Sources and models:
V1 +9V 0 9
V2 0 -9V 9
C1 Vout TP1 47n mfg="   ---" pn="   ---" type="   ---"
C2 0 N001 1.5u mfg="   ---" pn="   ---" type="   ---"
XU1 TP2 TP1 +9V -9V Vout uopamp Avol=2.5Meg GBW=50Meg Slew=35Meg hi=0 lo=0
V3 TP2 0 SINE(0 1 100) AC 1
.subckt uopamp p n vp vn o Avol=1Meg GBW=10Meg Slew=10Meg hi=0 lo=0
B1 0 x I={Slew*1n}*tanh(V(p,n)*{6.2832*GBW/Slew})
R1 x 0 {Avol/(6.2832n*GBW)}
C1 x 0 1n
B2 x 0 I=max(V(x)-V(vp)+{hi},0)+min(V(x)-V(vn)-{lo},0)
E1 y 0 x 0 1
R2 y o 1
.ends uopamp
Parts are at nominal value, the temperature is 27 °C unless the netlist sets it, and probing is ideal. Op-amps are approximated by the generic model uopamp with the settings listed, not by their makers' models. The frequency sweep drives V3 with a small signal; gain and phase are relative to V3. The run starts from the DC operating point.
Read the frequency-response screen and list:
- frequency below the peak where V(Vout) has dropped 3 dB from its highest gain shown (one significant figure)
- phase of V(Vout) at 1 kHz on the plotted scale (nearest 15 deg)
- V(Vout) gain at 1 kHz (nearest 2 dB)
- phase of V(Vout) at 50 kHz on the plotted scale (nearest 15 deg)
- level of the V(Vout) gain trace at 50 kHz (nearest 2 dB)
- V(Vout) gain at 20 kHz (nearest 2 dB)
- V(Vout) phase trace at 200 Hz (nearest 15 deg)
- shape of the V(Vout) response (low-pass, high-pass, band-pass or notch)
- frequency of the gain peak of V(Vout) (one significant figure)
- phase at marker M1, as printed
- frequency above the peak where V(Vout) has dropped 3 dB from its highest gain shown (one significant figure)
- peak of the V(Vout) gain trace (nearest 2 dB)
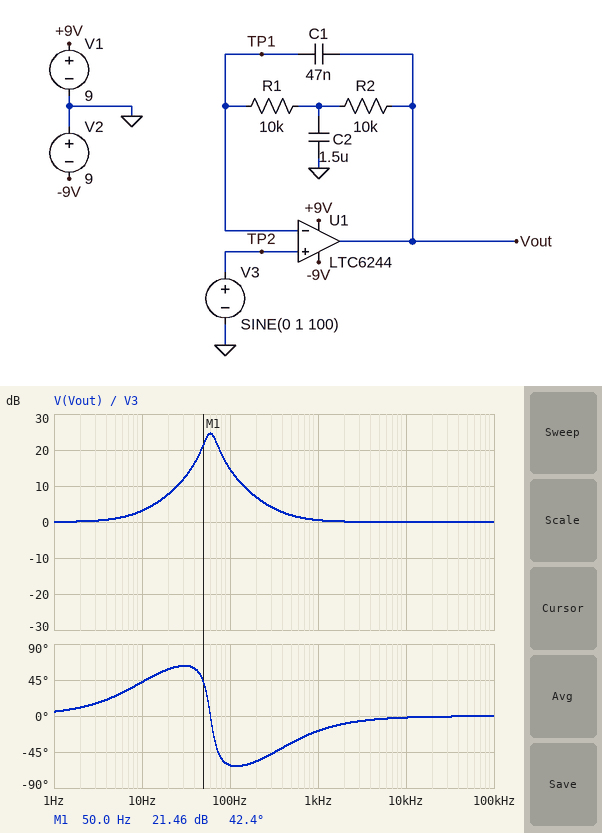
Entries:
50 Hz
-15 deg
0 dB
0 deg
0 dB
0 dB
-60 deg
band-pass
60 Hz
42.4 deg
70 Hz
24 dB
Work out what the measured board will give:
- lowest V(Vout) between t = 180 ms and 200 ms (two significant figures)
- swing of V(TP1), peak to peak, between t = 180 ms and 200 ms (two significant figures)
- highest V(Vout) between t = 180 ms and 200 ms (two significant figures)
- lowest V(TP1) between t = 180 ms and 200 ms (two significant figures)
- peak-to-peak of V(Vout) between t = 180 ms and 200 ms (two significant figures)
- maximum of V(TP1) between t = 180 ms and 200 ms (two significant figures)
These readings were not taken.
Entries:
-5.4 V
2.0 V
5.4 V
-1.0 V
11 V
1.0 V
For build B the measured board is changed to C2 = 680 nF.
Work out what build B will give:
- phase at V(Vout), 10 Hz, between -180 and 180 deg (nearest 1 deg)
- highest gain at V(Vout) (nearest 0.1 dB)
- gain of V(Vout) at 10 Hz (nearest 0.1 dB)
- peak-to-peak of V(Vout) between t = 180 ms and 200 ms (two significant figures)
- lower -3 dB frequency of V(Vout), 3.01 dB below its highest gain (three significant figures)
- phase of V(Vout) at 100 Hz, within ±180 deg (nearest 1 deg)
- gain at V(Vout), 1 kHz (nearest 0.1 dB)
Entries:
23 deg
18.3 dB
0.9 dB
15 V
68.4 Hz
-21 deg
0.6 dB
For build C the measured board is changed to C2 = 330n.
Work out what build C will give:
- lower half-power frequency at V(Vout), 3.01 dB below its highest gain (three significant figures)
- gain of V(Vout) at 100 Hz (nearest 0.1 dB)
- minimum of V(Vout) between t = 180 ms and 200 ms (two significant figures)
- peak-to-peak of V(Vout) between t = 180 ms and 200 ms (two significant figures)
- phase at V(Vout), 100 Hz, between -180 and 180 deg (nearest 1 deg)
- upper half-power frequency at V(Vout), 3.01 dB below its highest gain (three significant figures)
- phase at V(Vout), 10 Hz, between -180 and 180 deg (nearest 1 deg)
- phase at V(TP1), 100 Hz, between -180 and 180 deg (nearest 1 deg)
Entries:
86.7 Hz
11.6 dB
-3.8 V
7.6 V
25 deg
188 Hz
12 deg
0 deg
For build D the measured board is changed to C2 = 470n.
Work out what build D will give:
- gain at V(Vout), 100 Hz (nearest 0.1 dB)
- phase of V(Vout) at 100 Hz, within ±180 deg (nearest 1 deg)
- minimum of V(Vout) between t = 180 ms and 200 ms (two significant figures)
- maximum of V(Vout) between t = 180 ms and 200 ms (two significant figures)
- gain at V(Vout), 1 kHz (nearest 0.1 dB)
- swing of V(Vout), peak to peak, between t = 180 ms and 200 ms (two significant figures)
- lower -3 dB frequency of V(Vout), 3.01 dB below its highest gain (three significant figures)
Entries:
15.4 dB
10 deg
-5.9 V
5.9 V
0.7 dB
12 V
77.8 Hz
